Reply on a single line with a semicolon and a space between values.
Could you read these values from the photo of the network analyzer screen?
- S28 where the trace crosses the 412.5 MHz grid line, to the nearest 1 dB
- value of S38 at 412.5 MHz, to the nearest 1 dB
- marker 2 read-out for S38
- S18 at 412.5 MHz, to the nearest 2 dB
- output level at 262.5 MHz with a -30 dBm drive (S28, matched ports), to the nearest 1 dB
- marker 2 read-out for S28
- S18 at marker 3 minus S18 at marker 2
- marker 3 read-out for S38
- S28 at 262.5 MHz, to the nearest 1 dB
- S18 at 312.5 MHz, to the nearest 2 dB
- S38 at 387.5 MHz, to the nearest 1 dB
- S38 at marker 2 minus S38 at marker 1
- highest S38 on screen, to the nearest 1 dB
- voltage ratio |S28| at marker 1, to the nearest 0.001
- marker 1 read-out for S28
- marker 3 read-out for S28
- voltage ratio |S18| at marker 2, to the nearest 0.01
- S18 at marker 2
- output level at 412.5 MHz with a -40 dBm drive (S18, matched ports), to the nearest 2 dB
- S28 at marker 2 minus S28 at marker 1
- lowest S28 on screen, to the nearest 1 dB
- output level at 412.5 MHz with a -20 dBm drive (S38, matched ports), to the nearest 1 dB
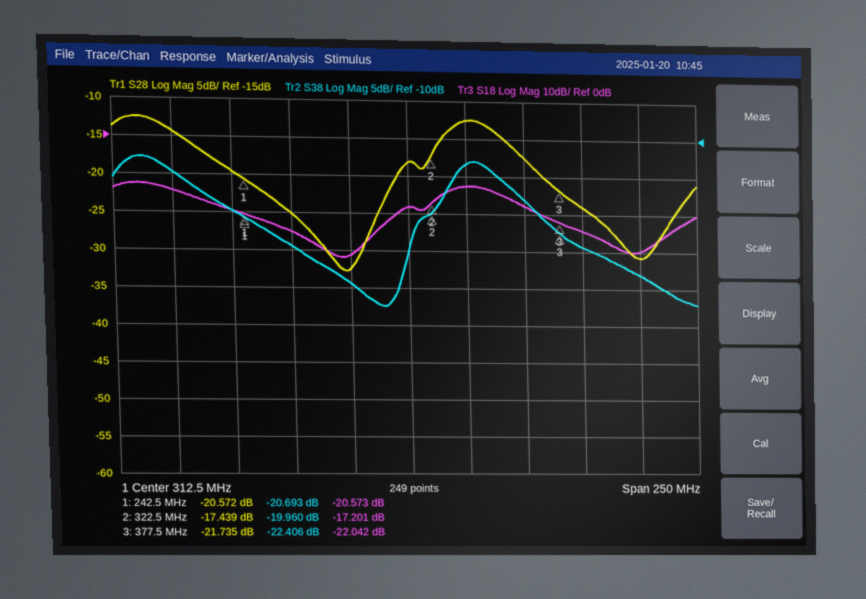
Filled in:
-31 dB; -28 dB; -19.960 dB; -30 dB; -55 dBm; -17.439 dB; -4.841 dB; -22.406 dB; -25 dB; -18 dB; -24 dB; 0.733 dB; -13 dB; 0.094; -20.572 dB; -21.735 dB; 0.14; -17.201 dB; -70 dBm; 3.133 dB; -33 dB; -48 dBm
